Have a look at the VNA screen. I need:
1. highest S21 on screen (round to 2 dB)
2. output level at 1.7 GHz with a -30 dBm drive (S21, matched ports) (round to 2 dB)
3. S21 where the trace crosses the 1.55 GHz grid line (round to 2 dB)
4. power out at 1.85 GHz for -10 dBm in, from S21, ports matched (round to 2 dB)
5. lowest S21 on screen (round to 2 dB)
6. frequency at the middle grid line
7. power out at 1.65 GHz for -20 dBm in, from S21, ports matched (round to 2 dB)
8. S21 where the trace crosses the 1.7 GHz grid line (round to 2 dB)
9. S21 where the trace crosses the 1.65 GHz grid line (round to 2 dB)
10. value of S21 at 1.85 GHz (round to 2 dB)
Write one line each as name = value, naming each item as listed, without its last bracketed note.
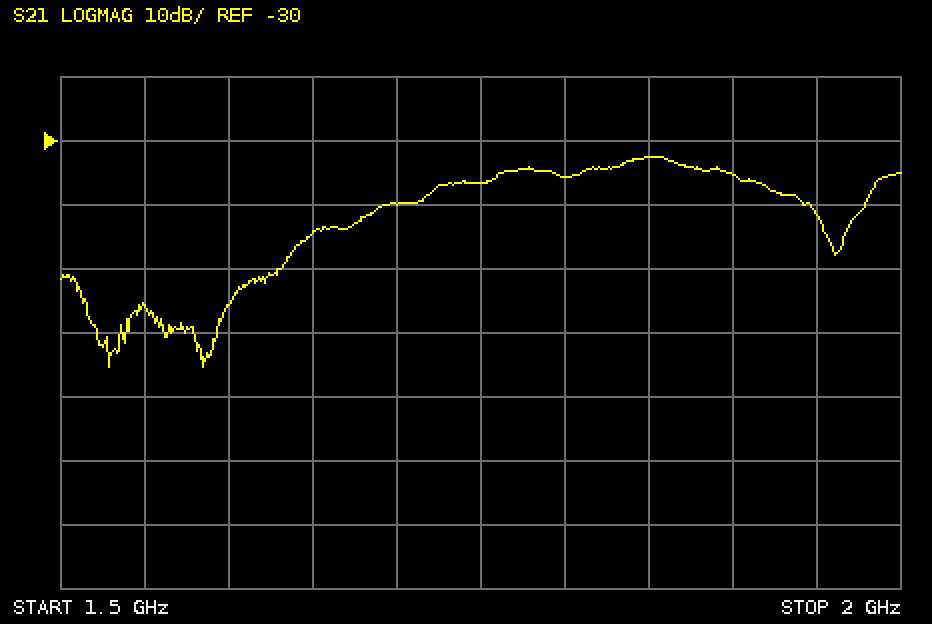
highest S21 on screen = -32 dB
output level at 1.7 GHz with a -30 dBm drive (S21, matched ports) = -70 dBm
S21 where the trace crosses the 1.55 GHz grid line = -56 dB
power out at 1.85 GHz for -10 dBm in, from S21, ports matched = -42 dBm
lowest S21 on screen = -66 dB
frequency at the middle grid line = 1.75 GHz
power out at 1.65 GHz for -20 dBm in, from S21, ports matched = -64 dBm
S21 where the trace crosses the 1.7 GHz grid line = -40 dB
S21 where the trace crosses the 1.65 GHz grid line = -44 dB
value of S21 at 1.85 GHz = -32 dB
